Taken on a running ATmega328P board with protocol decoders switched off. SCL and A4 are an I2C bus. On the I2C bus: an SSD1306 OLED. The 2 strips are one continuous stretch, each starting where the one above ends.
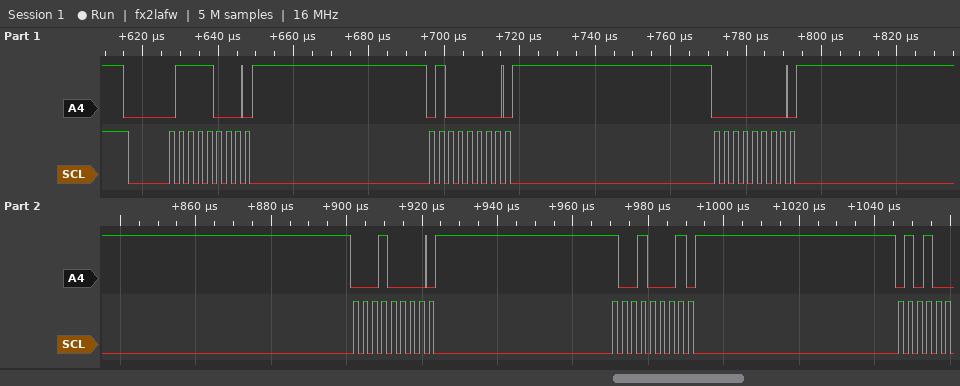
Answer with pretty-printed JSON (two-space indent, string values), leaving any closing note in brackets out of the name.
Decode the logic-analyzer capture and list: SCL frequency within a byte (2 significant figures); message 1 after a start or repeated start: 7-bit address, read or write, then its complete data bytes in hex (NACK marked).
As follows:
{
  "SCL frequency within a byte": "400 kHz",
  "message 1 after a start or repeated start: 7-bit address, read or write, then its complete data bytes in hex": "0x3C write: 40 00 10 91"
}
